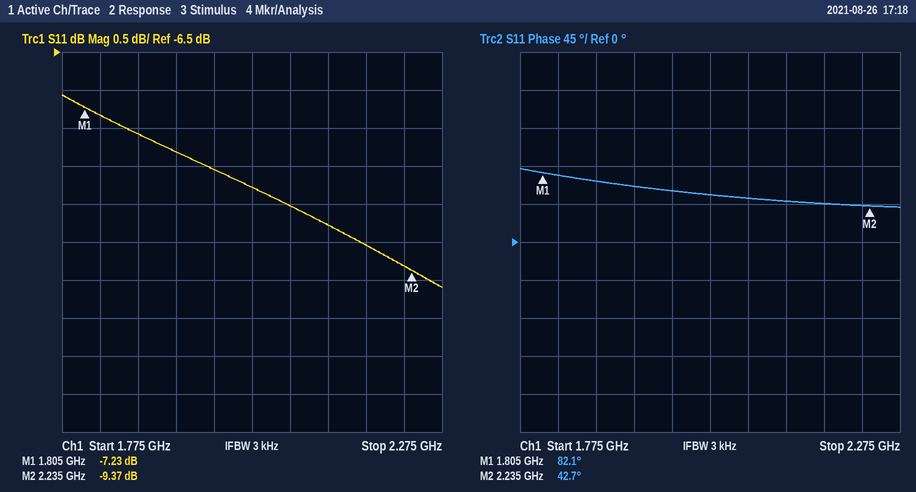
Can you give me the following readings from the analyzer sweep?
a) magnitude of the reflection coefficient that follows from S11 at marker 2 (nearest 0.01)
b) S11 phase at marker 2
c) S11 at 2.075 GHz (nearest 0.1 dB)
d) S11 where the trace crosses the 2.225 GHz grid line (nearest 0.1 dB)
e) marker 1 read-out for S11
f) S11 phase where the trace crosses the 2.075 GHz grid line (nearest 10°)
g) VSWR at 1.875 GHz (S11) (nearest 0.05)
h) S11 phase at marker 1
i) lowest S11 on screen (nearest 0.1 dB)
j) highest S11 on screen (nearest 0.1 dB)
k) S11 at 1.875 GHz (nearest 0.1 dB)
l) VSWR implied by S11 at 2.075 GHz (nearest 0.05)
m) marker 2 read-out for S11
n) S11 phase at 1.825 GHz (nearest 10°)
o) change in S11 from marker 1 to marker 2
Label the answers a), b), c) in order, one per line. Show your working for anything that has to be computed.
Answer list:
a) 10^(-9.37/20) ≈ 0.34
b) 42.7°
c) -8.5 dB
d) -9.3 dB
e) -7.23 dB
f) 50°
g) |Γ| = 10^(-7.6/20) = 0.4169; VSWR = (1 + 0.4169)/(1 − 0.4169) ≈ 2.43, so 2.45 to the nearest 0.05
h) 82.1°
i) -9.6 dB
j) -7.1 dB
k) -7.6 dB
l) |Γ| = 10^(-8.5/20) = 0.3758; VSWR = (1 + 0.3758)/(1 − 0.3758) ≈ 2.20
m) -9.37 dB
n) 80°
o) -9.37 − (-7.23) = -2.14 dB
